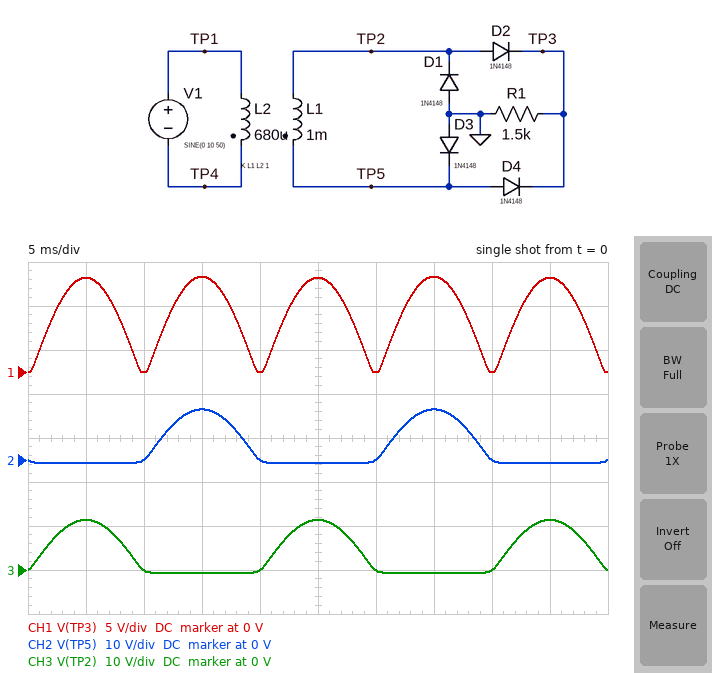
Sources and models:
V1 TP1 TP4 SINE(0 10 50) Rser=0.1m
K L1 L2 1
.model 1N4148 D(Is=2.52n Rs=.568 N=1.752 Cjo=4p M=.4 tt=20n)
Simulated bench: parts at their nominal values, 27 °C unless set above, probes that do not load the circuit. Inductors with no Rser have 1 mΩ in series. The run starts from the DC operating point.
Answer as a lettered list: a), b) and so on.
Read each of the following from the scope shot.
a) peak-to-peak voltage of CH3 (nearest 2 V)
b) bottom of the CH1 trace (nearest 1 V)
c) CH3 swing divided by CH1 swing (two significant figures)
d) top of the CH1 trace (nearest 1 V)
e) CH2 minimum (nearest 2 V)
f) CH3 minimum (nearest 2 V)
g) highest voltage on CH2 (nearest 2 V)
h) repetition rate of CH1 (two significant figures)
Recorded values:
a) 12 V
b) 0 V
c) 1.1
d) 11 V
e) 0 V
f) 0 V
g) 12 V
h) 100 Hz
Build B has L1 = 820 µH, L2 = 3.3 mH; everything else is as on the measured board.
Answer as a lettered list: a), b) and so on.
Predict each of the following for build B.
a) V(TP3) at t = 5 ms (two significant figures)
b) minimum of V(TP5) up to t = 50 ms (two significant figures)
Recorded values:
a) 3.7 V
b) -630 mV
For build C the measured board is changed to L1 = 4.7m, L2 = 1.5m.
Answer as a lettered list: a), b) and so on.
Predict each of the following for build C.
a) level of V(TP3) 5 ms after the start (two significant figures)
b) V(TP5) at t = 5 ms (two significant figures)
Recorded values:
a) 16 V
b) -700 mV
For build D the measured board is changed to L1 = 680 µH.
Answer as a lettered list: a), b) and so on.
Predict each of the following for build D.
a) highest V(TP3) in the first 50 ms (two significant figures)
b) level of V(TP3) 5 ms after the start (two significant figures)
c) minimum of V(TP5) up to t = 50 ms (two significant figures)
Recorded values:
a) 8.7 V
b) 8.6 V
c) -670 mV
